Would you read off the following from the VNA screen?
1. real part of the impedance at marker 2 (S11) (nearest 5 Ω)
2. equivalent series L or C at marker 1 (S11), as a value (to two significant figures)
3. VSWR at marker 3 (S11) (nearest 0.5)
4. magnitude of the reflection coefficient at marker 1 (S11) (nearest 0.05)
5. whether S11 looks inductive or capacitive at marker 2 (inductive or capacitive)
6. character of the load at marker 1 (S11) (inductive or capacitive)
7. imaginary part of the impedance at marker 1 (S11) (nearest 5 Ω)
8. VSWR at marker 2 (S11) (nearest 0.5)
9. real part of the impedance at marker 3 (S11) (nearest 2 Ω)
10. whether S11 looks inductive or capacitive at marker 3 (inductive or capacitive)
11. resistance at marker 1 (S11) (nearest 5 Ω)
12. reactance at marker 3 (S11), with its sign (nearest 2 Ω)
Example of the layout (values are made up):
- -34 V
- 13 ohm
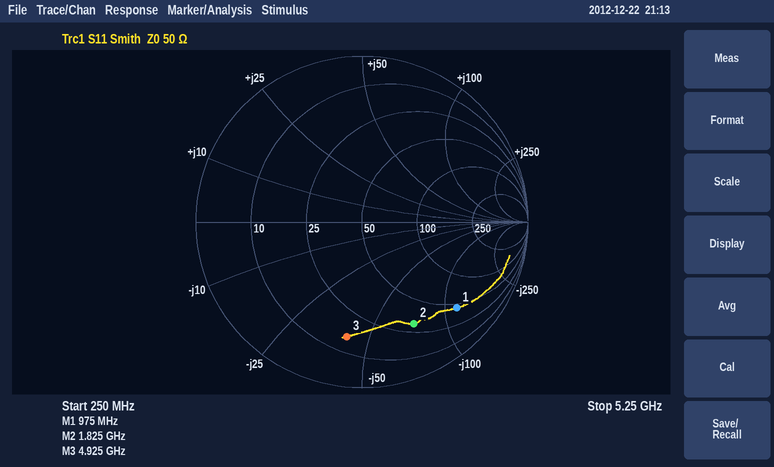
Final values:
- 30 Ω
- 1.4 pF
- 5.5
- 0.75
- capacitive
- capacitive
- -115 Ω
- 5.5
- 16 Ω
- capacitive
- 45 Ω
- -42 Ω
